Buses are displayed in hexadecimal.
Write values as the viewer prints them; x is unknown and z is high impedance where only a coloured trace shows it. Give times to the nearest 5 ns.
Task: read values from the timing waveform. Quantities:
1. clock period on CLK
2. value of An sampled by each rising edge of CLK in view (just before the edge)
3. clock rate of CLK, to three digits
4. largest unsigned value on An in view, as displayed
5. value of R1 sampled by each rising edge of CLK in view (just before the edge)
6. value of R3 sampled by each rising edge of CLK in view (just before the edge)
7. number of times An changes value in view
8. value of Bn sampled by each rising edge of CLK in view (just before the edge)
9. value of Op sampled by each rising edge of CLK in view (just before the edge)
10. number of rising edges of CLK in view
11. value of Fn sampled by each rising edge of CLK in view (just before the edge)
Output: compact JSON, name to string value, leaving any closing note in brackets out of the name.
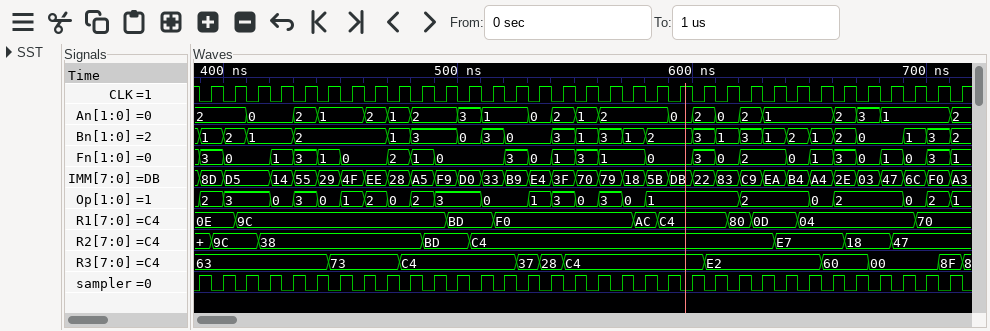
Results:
{"clock period on CLK": "10 ns", "value of An sampled by each rising edge of CLK in view": "2, 2, 0, 0, 2, 1, 1, 2, 1, 2, 2, 3, 1, 1, 0, 2, 1, 2, 2, 2, 0, 2, 0, 2, 1, 1, 1, 2, 3, 1, 1, 1, 2", "clock rate of CLK, to three digits": "100 MHz", "largest unsigned value on An in view, as displayed": "3", "value of R1 sampled by each rising edge of CLK in view": "0E, 0E, 9C, 9C, 9C, 9C, 9C, 9C, 9C, 9C, 9C, BD, BD, F0, F0, F0, F0, F0, F0, AC, C4, C4, C4, 80, 0D, 0D, 04, 04, 04, 04, 04, 70, 70", "value of R3 sampled by each rising edge of CLK in view": "63, 63, 63, 63, 63, 63, 73, 73, 73, C4, C4, C4, C4, C4, 37, 28, C4, C4, C4, C4, C4, C4, E2, E2, E2, E2, E2, 60, 60, 00, 00, 00, 8F", "number of times An changes value in view": "21", "value of Bn sampled by each rising edge of CLK in view": "1, 2, 1, 1, 2, 2, 2, 2, 1, 3, 3, 0, 3, 0, 0, 3, 1, 3, 1, 2, 2, 3, 1, 3, 1, 2, 1, 2, 0, 0, 1, 3, 2", "value of Op sampled by each rising edge of CLK in view": "2, 3, 3, 0, 3, 0, 1, 2, 0, 2, 3, 3, 0, 0, 1, 3, 0, 3, 0, 1, 1, 1, 1, 2, 2, 2, 0, 2, 2, 2, 0, 2, 1", "number of rising edges of CLK in view": "33", "value of Fn sampled by each rising edge of CLK in view": "3, 0, 0, 1, 3, 1, 0, 0, 2, 1, 0, 0, 0, 3, 0, 1, 3, 1, 1, 0, 0, 3, 0, 2, 2, 0, 1, 3, 0, 1, 0, 3, 1"}
